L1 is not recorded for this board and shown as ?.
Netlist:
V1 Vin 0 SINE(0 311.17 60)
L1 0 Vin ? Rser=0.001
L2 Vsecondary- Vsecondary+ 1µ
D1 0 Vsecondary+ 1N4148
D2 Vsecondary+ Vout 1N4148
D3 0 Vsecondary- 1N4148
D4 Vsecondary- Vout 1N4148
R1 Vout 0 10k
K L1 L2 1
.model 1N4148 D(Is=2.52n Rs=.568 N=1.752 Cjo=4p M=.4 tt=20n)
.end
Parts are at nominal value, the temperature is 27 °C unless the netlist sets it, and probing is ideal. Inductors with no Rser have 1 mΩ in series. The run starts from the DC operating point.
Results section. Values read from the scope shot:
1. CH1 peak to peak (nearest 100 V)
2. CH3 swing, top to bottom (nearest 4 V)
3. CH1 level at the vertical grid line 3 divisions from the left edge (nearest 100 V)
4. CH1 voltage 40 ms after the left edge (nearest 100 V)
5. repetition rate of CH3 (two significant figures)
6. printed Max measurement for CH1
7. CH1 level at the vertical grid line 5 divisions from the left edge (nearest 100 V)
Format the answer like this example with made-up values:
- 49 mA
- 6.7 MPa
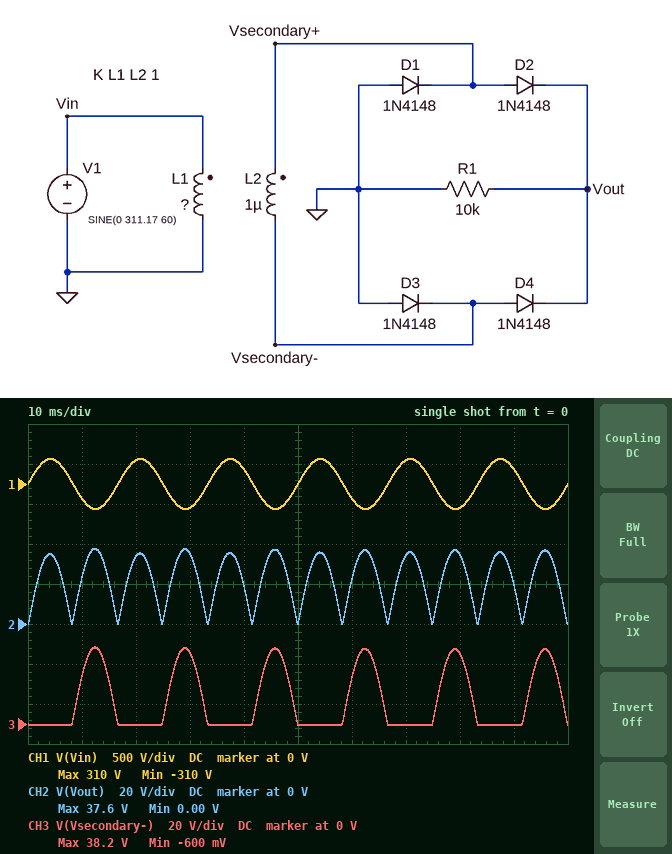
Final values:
- 600 V
- 40 V
- -300 V
- 200 V
- 60 Hz
- 310 V
- 0 V
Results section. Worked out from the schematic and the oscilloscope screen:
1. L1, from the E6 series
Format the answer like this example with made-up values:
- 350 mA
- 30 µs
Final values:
- 68 µH
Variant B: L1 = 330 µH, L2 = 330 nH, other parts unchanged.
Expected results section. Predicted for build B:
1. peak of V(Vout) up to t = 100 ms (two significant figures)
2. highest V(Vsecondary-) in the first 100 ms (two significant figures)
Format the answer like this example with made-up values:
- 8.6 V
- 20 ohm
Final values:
- 8.8 V
- 9.3 V
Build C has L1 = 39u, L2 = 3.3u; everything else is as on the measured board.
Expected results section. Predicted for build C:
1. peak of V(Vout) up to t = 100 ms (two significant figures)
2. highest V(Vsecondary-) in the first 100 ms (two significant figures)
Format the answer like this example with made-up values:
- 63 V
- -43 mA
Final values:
- 93 V
- 94 V
